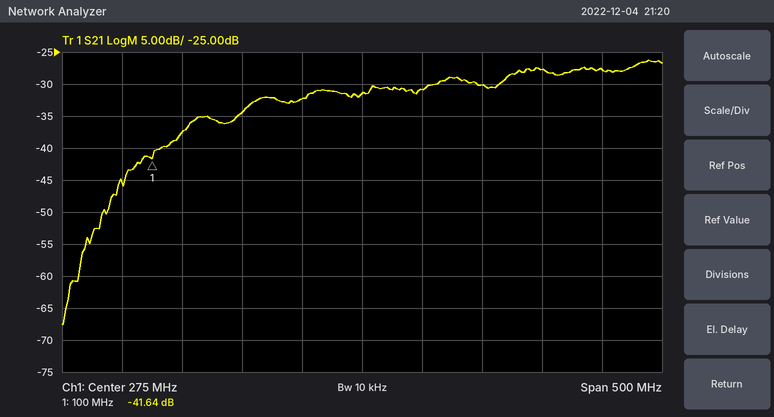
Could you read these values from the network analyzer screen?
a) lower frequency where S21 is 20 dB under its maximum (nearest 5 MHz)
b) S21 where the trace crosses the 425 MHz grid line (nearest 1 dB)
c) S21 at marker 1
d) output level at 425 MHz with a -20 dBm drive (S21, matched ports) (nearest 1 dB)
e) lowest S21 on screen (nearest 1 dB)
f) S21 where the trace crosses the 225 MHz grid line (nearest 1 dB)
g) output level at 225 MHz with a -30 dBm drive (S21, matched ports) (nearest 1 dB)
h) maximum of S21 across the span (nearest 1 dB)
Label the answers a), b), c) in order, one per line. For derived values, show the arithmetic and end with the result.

a) 70 MHz
b) -28 dB
c) -41.64 dB
d) -20 dBm + (-28 dB) = -48 dBm
e) -68 dB
f) -32 dB
g) -30 dBm + (-32 dB) = -62 dBm
h) -26 dB
